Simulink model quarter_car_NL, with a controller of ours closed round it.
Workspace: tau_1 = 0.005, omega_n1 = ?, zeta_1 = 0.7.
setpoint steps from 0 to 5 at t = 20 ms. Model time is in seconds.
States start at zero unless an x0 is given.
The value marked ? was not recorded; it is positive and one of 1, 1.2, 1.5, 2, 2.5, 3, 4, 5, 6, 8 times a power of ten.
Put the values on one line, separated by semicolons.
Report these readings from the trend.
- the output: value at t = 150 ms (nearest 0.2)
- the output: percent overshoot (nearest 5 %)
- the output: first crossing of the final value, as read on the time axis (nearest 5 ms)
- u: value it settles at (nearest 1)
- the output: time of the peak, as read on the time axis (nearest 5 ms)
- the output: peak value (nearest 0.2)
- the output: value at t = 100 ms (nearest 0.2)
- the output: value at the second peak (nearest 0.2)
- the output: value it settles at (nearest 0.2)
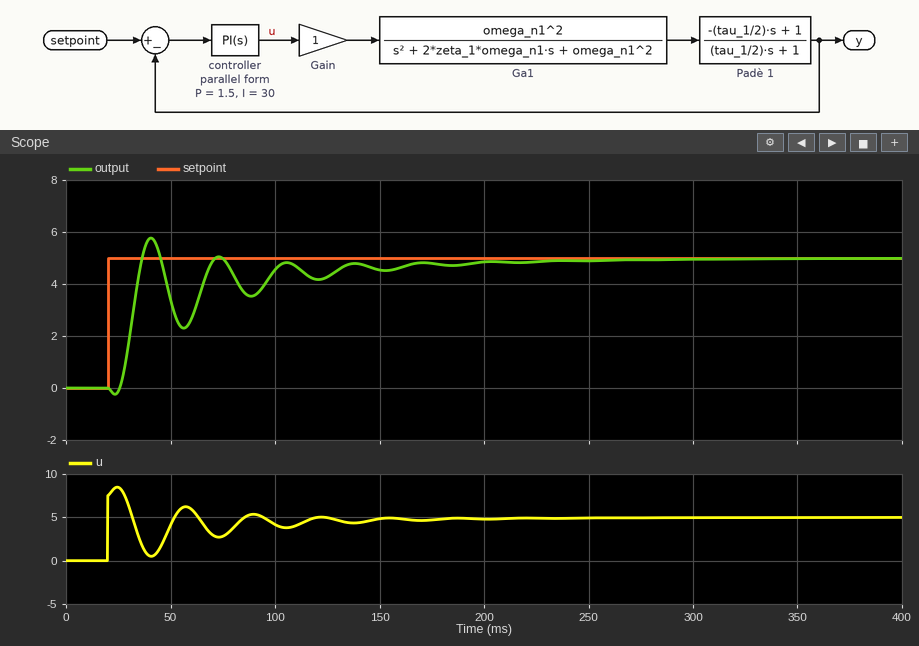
4.6; 15 %; 35 ms; 5; 40 ms; 5.8; 4.6; 5.0; 5.0
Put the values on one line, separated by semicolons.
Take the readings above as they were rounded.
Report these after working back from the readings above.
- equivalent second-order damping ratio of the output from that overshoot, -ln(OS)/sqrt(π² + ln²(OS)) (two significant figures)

0.52
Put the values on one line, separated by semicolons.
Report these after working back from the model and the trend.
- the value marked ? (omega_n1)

150
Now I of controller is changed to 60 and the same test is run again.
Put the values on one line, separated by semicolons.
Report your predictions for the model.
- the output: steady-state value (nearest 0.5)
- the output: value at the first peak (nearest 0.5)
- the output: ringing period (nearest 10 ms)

5.0; 6.5; 30 ms
